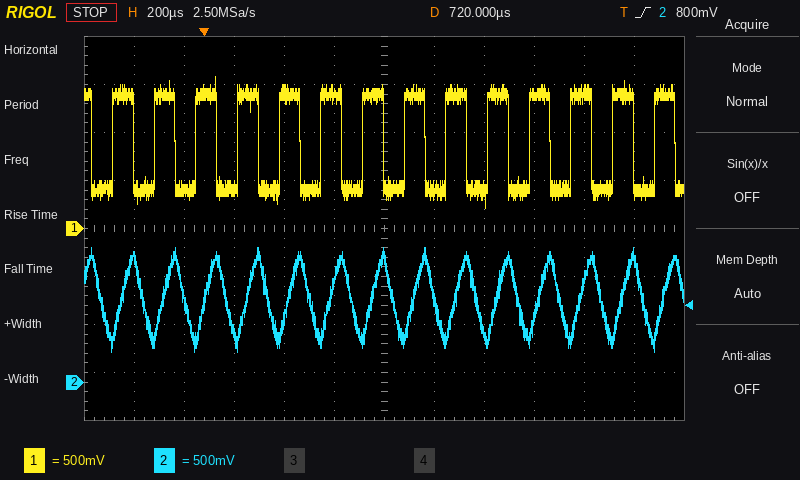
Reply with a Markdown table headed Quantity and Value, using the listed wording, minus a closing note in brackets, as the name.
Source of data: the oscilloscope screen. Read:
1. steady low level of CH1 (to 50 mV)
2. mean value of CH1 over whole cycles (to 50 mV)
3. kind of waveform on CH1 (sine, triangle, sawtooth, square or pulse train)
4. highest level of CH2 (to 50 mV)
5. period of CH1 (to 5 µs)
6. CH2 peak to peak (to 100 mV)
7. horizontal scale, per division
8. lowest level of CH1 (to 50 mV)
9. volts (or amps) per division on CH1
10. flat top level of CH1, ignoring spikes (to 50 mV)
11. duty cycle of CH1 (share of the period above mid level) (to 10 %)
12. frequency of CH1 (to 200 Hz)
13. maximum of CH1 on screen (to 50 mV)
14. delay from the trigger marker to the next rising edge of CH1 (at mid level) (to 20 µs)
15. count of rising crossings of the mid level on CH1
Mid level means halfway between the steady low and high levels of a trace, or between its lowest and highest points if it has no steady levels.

| Quantity | Value |
|---|---|
| steady low level of CH1 | 400 mV |
| mean value of CH1 over whole cycles | 900 mV |
| kind of waveform on CH1 | square |
| highest level of CH2 | 1.40 V |
| period of CH1 | 165 µs |
| CH2 peak to peak | 1.10 V |
| horizontal scale, per division | 200 µs |
| lowest level of CH1 | 200 mV |
| volts (or amps) per division on CH1 | 500 mV |
| flat top level of CH1, ignoring spikes | 1.40 V |
| duty cycle of CH1 (share of the period above mid level) | 50 % |
| frequency of CH1 | 6.0 kHz |
| maximum of CH1 on screen | 1.60 V |
| delay from the trigger marker to the next rising edge of CH1 (at mid level) | 140 µs |
| count of rising crossings of the mid level on CH1 | 14 |
